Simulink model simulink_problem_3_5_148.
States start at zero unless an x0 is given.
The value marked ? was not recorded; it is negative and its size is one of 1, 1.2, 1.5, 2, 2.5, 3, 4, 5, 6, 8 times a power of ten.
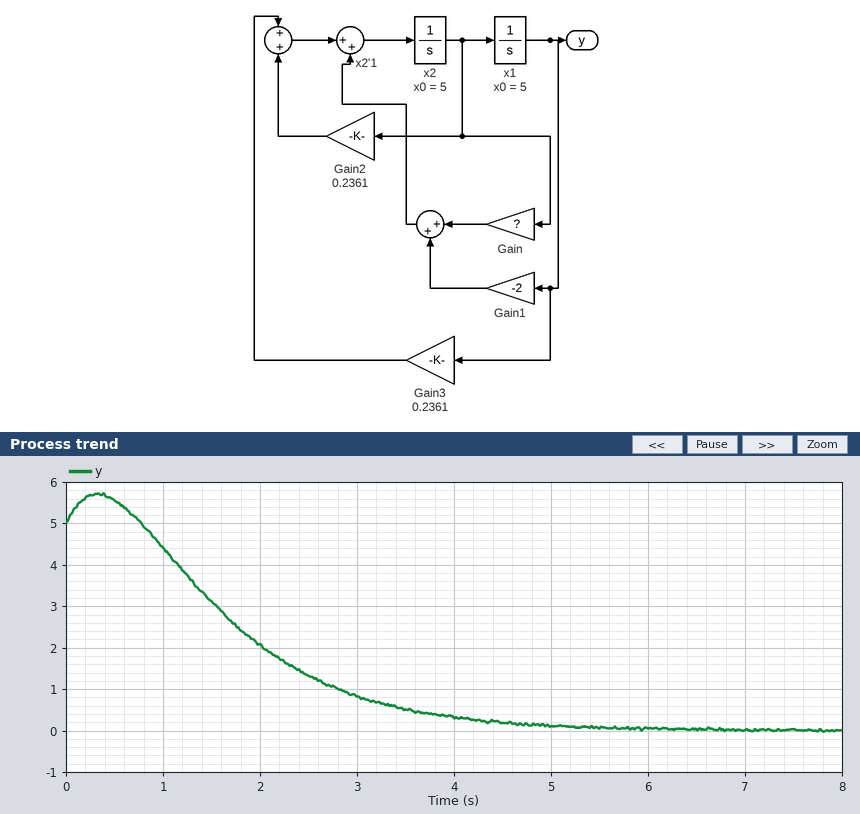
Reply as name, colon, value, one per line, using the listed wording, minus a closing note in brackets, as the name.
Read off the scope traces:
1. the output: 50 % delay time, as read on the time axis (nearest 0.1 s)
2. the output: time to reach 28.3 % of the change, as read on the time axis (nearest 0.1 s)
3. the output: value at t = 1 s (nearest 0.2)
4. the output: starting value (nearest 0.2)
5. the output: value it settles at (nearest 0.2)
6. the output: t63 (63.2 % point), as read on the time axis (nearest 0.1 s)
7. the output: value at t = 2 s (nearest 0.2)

the output: 50 % delay time, as read on the time axis: 1.8 s
the output: time to reach 28.3 % of the change, as read on the time axis: 1.3 s
the output: value at t = 1 s: 4.4
the output: starting value: 5.0
the output: value it settles at: 0.0
the output: t63 (63.2 % point), as read on the time axis: 2.1 s
the output: value at t = 2 s: 2.0
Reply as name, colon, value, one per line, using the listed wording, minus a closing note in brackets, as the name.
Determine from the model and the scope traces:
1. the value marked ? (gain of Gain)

the value marked ?: -3
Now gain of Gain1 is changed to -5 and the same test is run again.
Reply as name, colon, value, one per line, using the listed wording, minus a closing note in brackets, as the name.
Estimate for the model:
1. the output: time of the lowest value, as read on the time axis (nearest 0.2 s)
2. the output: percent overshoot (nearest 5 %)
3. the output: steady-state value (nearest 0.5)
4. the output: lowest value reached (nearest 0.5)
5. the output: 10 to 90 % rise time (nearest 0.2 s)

the output: time of the lowest value, as read on the time axis: 2.0 s
the output: percent overshoot: 10 %
the output: steady-state value: 0.0
the output: lowest value reached: -0.5
the output: 10 to 90 % rise time: 0.8 s
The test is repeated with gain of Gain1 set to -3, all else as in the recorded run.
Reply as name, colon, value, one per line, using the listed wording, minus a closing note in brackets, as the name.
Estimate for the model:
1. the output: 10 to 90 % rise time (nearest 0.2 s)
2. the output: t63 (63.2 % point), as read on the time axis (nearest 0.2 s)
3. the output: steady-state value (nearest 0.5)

the output: 10 to 90 % rise time: 1.4 s
the output: t63 (63.2 % point), as read on the time axis: 1.4 s
the output: steady-state value: 0.0
